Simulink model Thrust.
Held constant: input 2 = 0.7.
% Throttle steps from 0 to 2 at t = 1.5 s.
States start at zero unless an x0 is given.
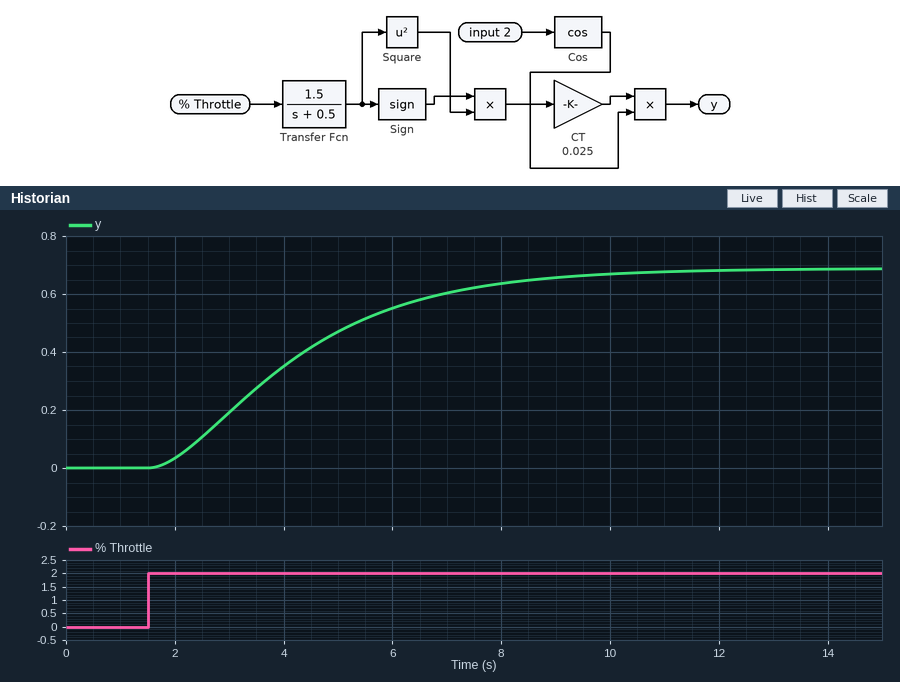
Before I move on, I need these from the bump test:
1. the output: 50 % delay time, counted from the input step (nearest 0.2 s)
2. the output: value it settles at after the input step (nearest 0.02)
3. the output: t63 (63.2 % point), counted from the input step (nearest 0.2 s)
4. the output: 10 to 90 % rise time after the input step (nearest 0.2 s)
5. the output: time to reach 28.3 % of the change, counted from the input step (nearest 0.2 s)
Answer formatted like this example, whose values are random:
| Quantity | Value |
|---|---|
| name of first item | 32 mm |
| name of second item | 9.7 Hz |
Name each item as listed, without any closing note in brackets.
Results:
| Quantity | Value |
|---|---|
| the output: 50 % delay time, counted from the input step | 2.4 s |
| the output: value it settles at after the input step | 0.68 |
| the output: t63 (63.2 % point), counted from the input step | 3.2 s |
| the output: 10 to 90 % rise time after the input step | 5.2 s |
| the output: time to reach 28.3 % of the change, counted from the input step | 1.6 s |
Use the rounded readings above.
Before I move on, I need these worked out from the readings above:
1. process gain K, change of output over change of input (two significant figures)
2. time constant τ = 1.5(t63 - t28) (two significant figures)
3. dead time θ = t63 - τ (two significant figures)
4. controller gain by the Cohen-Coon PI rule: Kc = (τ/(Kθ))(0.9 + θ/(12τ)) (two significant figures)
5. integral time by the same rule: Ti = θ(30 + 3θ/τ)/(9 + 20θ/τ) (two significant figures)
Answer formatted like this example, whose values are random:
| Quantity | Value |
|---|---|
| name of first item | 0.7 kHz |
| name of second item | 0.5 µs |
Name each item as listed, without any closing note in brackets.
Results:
| Quantity | Value |
|---|---|
| process gain K, change of output over change of input | 0.34 |
| time constant τ = 1.5(t63 - t28) | 2.4 s |
| dead time θ = t63 - τ | 0.80 s |
| controller gain by the Cohen-Coon PI rule: Kc = (τ/(Kθ))(0.9 + θ/(12τ)) | 8.2 |
| integral time by the same rule: Ti = θ(30 + 3θ/τ)/(9 + 20θ/τ) | 1.6 s |
